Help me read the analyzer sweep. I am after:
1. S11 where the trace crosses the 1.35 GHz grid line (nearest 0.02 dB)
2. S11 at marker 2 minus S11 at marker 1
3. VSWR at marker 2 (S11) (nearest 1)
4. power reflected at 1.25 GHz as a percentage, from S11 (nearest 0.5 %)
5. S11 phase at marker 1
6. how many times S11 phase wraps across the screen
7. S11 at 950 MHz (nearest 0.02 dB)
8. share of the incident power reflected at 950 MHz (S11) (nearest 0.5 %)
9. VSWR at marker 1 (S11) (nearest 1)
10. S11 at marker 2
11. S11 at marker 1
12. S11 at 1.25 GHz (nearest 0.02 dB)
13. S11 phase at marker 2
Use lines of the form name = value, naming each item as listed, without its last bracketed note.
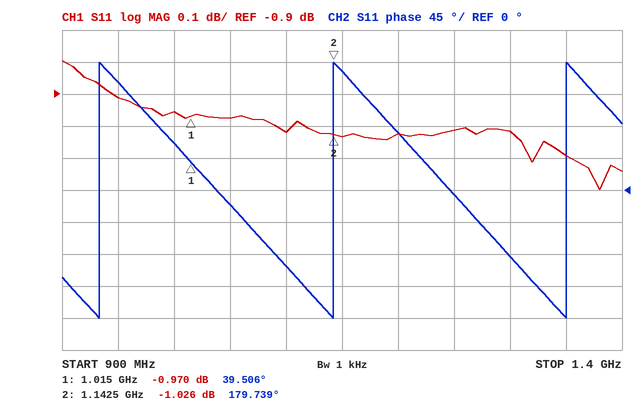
S11 where the trace crosses the 1.35 GHz grid line = -1.10 dB
S11 at marker 2 minus S11 at marker 1 = -0.056 dB
VSWR at marker 2 (S11) = 17
power reflected at 1.25 GHz as a percentage, from S11 = 79.0 %
S11 phase at marker 1 = 39.506°
how many times S11 phase wraps across the screen = 3
S11 at 950 MHz = -0.92 dB
share of the incident power reflected at 950 MHz (S11) = 81.0 %
VSWR at marker 1 (S11) = 18
S11 at marker 2 = -1.026 dB
S11 at marker 1 = -0.970 dB
S11 at 1.25 GHz = -1.02 dB
S11 phase at marker 2 = 179.739°
